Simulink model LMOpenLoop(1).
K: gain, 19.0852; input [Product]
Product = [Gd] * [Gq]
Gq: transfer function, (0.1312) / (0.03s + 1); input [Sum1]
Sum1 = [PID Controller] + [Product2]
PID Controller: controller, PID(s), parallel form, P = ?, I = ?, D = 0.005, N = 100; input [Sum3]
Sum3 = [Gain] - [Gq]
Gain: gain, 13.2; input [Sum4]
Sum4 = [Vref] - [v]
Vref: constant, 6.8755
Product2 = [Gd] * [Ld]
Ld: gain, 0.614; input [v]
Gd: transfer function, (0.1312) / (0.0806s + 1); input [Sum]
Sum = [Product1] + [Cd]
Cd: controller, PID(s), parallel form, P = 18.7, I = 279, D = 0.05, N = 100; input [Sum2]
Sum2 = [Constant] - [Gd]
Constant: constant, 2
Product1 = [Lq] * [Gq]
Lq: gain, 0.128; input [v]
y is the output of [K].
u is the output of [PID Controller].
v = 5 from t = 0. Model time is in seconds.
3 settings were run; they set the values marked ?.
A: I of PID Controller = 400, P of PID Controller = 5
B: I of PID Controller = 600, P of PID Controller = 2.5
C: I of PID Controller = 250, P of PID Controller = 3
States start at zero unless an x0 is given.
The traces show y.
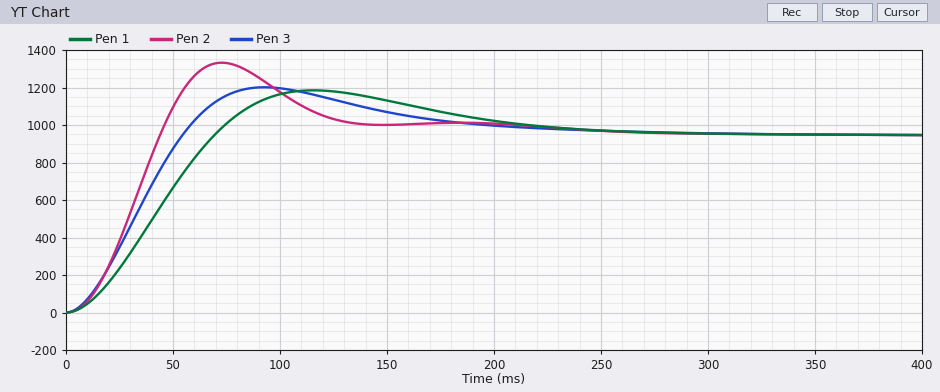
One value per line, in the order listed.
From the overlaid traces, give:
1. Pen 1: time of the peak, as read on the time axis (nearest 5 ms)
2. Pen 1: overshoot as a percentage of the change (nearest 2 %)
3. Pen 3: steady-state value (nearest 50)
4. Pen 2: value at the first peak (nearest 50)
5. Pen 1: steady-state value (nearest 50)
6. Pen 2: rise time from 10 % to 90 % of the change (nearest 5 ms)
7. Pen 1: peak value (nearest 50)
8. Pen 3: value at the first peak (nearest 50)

115 ms
26 %
950
1350
950
30 ms
1200
1200
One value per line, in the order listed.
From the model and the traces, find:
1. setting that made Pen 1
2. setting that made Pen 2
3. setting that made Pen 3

C
B
A
